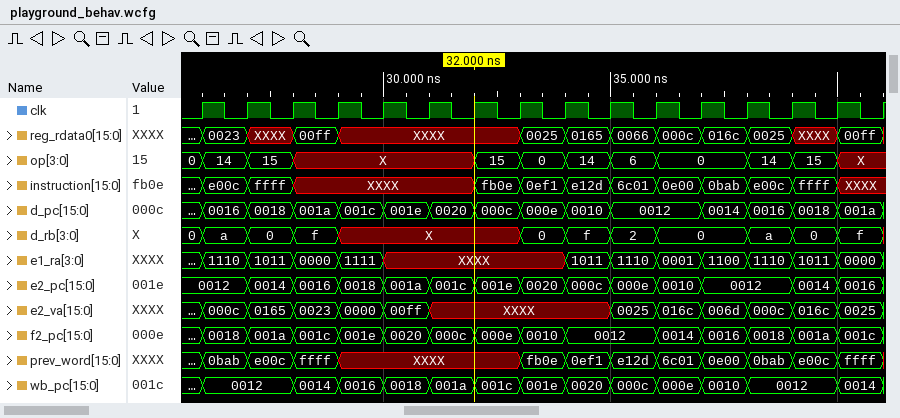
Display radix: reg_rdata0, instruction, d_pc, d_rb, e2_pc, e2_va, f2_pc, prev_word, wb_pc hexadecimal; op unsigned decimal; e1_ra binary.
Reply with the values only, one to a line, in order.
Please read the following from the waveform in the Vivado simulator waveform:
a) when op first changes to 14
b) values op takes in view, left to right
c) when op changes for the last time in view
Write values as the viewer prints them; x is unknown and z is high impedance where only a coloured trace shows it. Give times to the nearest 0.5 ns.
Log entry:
26 ns
0, 14, 15, X, 15, 0, 14, 6, 0, 14, 15, X
40 ns
